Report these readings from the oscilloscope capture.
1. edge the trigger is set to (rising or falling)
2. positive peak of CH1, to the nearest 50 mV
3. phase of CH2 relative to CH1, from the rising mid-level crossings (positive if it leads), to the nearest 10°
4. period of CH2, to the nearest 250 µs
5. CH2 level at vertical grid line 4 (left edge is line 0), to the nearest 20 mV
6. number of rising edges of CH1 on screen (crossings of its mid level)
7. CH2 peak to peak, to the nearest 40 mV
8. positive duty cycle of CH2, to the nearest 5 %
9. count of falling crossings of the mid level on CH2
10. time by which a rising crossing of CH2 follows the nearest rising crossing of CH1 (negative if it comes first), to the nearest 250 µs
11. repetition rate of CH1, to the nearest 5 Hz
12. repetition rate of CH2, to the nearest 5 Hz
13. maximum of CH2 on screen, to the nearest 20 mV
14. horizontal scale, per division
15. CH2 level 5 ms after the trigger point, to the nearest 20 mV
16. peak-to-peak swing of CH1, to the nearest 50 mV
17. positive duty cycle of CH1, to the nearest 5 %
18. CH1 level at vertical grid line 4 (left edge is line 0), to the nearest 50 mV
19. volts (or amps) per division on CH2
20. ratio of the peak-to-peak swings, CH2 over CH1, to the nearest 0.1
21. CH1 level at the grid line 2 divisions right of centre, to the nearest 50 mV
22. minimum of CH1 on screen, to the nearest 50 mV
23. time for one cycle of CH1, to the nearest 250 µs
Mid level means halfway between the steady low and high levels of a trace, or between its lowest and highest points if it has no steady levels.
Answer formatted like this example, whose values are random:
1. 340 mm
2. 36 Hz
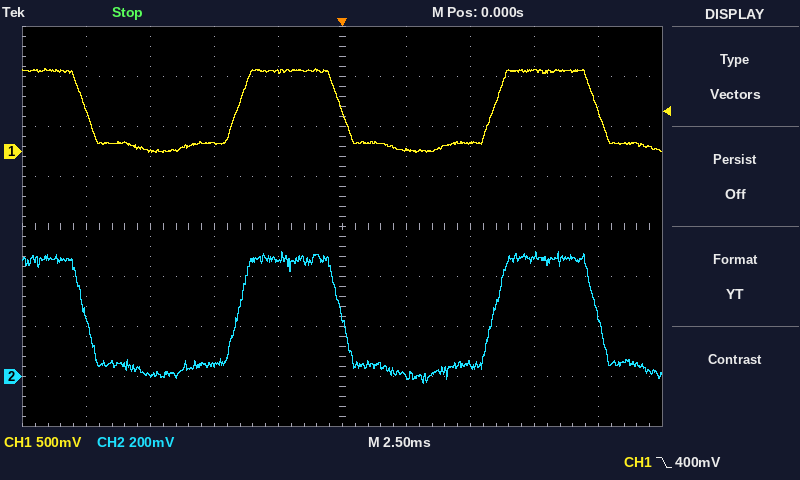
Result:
1. falling
2. 850 mV
3. 0°
4. 10.00 ms
5. 460 mV
6. 2
7. 520 mV
8. 40 %
9. 3
10. 0.00 ms
11. 100 Hz
12. 100 Hz
13. 500 mV
14. 2.5 ms
15. 40 mV
16. 850 mV
17. 40 %
18. 800 mV
19. 200 mV
20. 0.6
21. 100 mV
22. 0 mV
23. 10.00 ms
